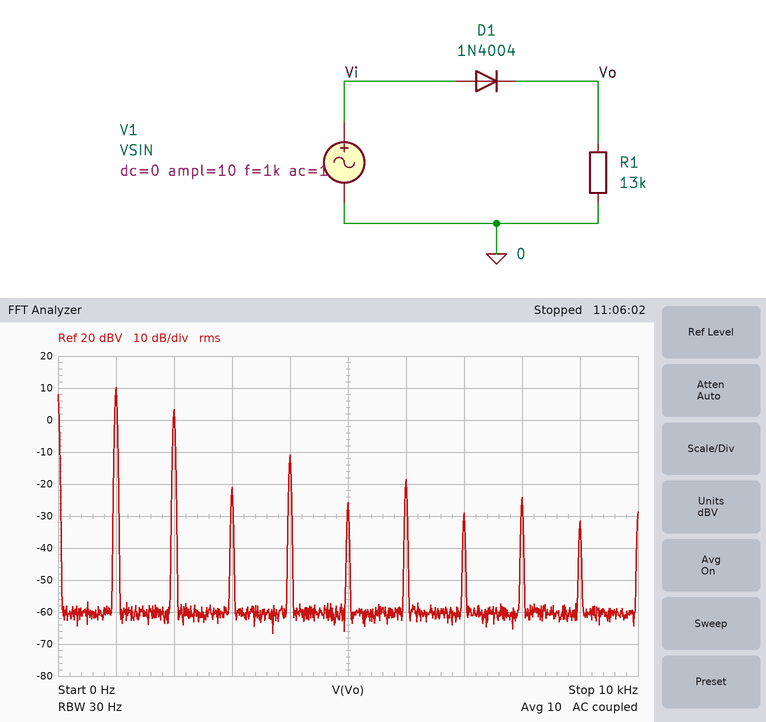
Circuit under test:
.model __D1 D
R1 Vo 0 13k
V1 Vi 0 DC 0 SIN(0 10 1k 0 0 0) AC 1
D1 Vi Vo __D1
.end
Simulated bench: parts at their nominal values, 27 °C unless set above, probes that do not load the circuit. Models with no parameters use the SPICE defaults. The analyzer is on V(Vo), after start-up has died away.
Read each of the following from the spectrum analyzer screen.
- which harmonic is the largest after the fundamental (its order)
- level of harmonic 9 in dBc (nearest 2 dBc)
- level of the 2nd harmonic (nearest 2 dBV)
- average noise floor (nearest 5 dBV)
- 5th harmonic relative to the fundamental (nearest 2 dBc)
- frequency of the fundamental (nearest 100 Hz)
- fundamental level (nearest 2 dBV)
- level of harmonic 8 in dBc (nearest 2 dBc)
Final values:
2
-42 dBc
4 dBV
-60 dBV
-36 dBc
1.0 kHz
10 dBV
-34 dBc
